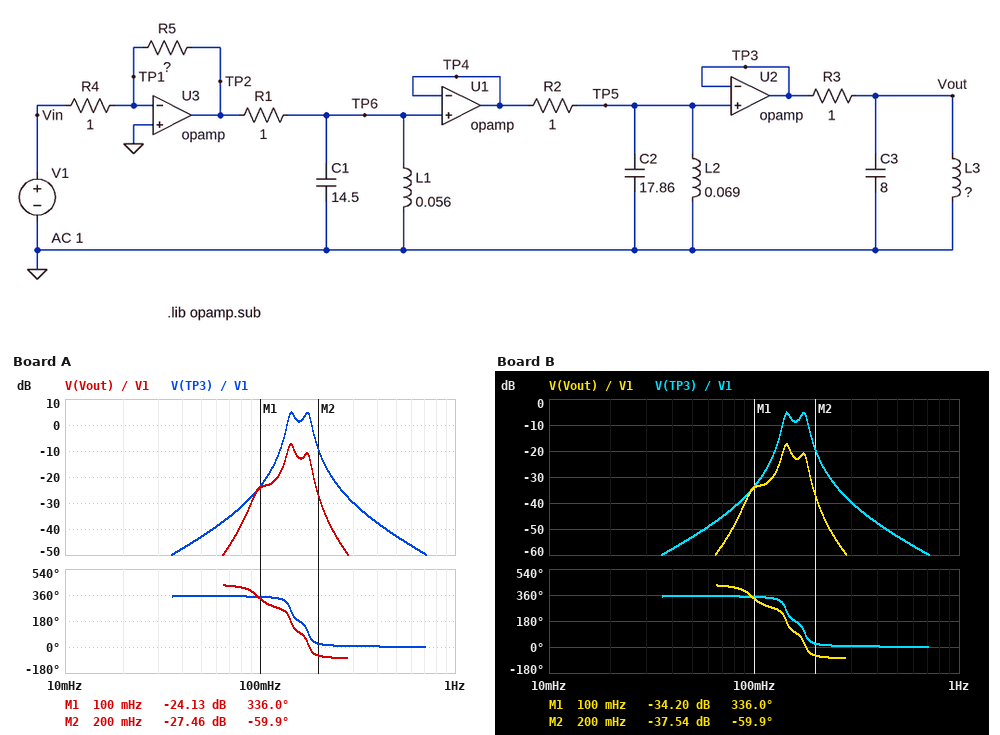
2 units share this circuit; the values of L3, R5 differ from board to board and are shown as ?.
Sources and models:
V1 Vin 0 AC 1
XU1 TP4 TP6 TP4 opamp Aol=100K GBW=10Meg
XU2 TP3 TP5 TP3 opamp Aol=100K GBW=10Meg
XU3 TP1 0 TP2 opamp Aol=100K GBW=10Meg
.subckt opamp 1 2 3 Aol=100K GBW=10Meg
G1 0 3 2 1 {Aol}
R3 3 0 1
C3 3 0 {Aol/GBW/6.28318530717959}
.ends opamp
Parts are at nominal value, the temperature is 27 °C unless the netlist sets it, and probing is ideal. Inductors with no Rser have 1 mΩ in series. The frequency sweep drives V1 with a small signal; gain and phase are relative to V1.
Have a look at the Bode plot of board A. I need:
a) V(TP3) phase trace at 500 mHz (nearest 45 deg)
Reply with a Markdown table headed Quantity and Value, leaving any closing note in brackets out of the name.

| Quantity | Value |
|---|---|
| V(TP3) phase trace at 500 mHz | 0 deg |
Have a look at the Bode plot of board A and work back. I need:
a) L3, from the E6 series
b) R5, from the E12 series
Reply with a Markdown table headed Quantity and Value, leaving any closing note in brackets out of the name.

| Quantity | Value |
|---|---|
| L3, from the E6 series | 330 mH |
| R5, from the E12 series | 15 Ω |
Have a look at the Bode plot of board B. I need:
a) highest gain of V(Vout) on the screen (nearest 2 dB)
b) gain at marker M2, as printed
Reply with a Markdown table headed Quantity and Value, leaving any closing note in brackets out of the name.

| Quantity | Value |
|---|---|
| highest gain of V(Vout) on the screen | -18 dB |
| gain at marker M2, as printed | -37.54 dB |
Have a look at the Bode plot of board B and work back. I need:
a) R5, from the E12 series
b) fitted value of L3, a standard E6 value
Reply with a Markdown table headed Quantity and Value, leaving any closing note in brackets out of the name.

| Quantity | Value |
|---|---|
| R5, from the E12 series | 4.7 Ω |
| fitted value of L3, a standard E6 value | 330 mH |
